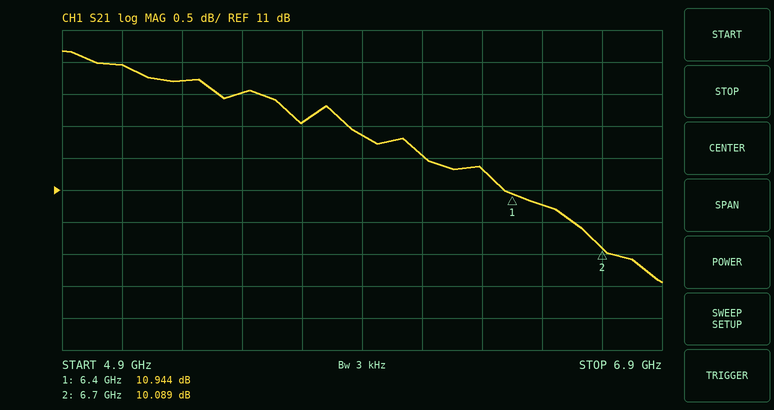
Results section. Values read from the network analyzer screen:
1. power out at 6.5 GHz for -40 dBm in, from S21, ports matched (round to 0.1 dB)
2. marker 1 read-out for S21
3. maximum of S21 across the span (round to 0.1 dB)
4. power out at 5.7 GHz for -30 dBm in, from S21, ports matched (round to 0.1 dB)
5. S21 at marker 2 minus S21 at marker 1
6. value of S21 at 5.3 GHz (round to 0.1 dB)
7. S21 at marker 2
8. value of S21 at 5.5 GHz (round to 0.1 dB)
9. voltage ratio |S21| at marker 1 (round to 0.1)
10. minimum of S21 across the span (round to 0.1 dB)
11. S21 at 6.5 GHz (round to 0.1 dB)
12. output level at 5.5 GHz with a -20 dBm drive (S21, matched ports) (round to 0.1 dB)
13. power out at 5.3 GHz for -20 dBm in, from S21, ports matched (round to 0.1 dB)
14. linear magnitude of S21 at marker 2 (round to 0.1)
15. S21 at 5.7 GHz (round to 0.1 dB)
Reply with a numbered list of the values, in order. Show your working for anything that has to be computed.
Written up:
1. -40 dBm + (10.8 dB) = -29.2 dBm
2. 10.944 dB
3. 13.2 dB
4. -30 dBm + (12.1 dB) = -17.9 dBm
5. 10.089 − (10.944) = -0.855 dB
6. 12.7 dB
7. 10.089 dB
8. 12.5 dB
9. 10^(10.944/20) ≈ 3.5
10. 9.6 dB
11. 10.8 dB
12. -20 dBm + (12.5 dB) = -7.5 dBm
13. -20 dBm + (12.7 dB) = -7.3 dBm
14. 10^(10.089/20) ≈ 3.2
15. 12.1 dB
